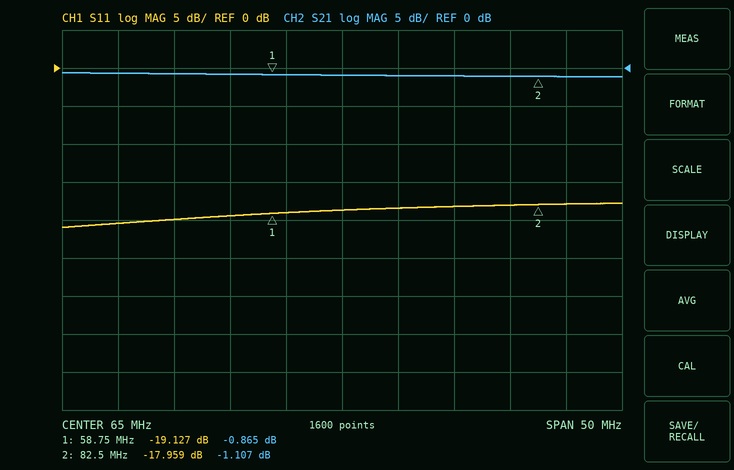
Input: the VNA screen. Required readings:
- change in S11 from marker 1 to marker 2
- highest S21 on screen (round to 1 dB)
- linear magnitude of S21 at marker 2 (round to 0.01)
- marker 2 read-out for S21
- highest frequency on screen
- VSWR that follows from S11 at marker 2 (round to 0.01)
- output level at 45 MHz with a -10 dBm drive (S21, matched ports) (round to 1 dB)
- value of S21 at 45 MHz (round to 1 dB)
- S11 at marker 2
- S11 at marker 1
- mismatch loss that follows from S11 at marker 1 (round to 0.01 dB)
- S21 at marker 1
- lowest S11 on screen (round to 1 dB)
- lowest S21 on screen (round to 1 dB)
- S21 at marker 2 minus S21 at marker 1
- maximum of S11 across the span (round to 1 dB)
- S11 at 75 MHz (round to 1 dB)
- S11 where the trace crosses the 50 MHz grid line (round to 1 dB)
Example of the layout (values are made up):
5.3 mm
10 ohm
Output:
1.168 dB
-1 dB
0.88
-1.107 dB
90 MHz
1.29
-11 dBm
-1 dB
-17.959 dB
-19.127 dB
0.05 dB
-0.865 dB
-21 dB
-1 dB
-0.242 dB
-18 dB
-18 dB
-20 dB
